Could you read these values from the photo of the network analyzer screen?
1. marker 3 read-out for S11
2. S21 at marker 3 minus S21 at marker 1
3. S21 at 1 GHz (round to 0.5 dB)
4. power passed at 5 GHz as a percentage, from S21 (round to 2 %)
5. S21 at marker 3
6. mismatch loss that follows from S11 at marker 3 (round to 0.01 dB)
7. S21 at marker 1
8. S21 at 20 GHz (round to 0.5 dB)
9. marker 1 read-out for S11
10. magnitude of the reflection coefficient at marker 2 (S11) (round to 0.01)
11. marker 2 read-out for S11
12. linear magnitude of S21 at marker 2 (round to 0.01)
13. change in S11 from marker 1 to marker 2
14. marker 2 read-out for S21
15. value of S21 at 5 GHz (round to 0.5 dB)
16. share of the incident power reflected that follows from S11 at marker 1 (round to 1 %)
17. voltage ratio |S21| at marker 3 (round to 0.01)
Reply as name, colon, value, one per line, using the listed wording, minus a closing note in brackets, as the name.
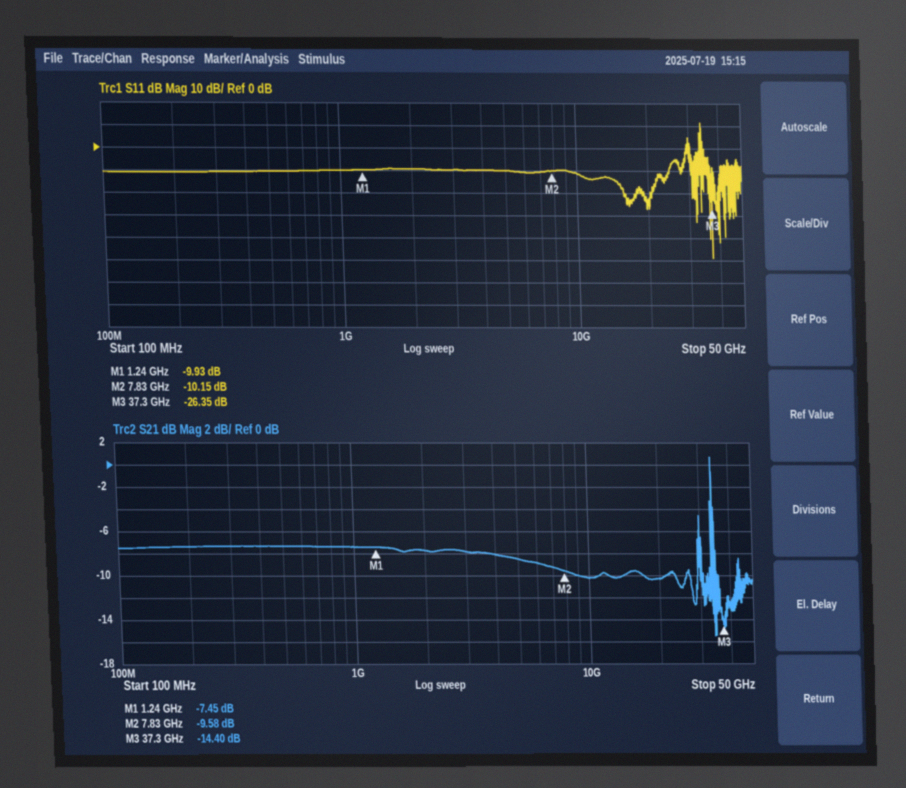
marker 3 read-out for S11: -26.35 dB
S21 at marker 3 minus S21 at marker 1: -6.95 dB
S21 at 1 GHz: -7.5 dB
power passed at 5 GHz as a percentage, from S21: 14 %
S21 at marker 3: -14.40 dB
mismatch loss that follows from S11 at marker 3: 0.01 dB
S21 at marker 1: -7.45 dB
S21 at 20 GHz: -10.5 dB
marker 1 read-out for S11: -9.93 dB
magnitude of the reflection coefficient at marker 2 (S11): 0.31
marker 2 read-out for S11: -10.15 dB
linear magnitude of S21 at marker 2: 0.33
change in S11 from marker 1 to marker 2: -0.22 dB
marker 2 read-out for S21: -9.58 dB
value of S21 at 5 GHz: -8.5 dB
share of the incident power reflected that follows from S11 at marker 1: 10 %
voltage ratio |S21| at marker 3: 0.19
